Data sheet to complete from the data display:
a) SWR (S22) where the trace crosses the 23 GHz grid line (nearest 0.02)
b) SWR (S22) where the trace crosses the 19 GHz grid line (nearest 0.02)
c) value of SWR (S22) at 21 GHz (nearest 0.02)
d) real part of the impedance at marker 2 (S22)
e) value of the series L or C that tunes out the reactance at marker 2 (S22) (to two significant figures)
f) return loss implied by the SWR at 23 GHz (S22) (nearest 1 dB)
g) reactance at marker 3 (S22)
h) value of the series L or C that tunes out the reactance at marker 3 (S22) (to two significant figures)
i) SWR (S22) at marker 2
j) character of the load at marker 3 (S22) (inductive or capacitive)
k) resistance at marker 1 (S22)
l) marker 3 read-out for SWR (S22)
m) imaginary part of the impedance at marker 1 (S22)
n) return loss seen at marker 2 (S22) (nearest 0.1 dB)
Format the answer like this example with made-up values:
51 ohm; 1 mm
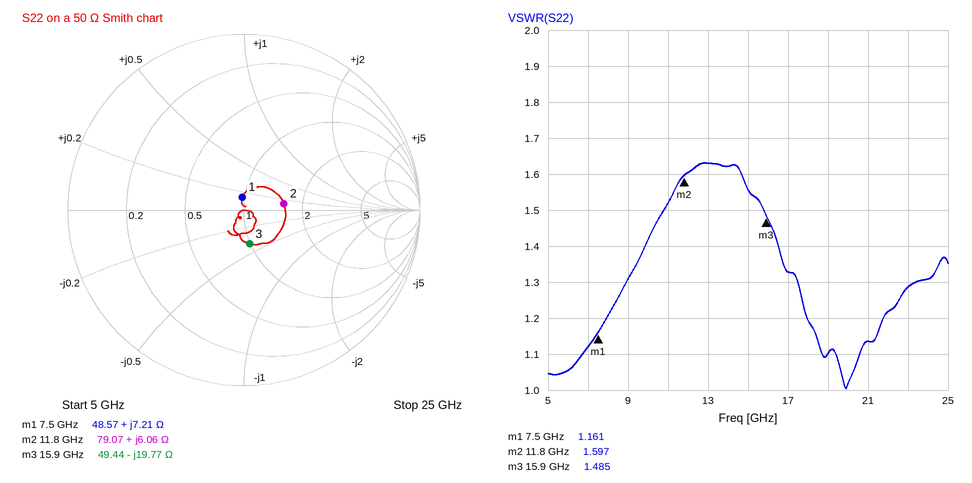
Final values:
1.28; 1.10; 1.14; 79.07 Ω; 2.2 pF; 18 dB; -19.77 Ω; 200 pH; 1.597; capacitive; 48.57 Ω; 1.485; +7.21 Ω; 12.8 dB
